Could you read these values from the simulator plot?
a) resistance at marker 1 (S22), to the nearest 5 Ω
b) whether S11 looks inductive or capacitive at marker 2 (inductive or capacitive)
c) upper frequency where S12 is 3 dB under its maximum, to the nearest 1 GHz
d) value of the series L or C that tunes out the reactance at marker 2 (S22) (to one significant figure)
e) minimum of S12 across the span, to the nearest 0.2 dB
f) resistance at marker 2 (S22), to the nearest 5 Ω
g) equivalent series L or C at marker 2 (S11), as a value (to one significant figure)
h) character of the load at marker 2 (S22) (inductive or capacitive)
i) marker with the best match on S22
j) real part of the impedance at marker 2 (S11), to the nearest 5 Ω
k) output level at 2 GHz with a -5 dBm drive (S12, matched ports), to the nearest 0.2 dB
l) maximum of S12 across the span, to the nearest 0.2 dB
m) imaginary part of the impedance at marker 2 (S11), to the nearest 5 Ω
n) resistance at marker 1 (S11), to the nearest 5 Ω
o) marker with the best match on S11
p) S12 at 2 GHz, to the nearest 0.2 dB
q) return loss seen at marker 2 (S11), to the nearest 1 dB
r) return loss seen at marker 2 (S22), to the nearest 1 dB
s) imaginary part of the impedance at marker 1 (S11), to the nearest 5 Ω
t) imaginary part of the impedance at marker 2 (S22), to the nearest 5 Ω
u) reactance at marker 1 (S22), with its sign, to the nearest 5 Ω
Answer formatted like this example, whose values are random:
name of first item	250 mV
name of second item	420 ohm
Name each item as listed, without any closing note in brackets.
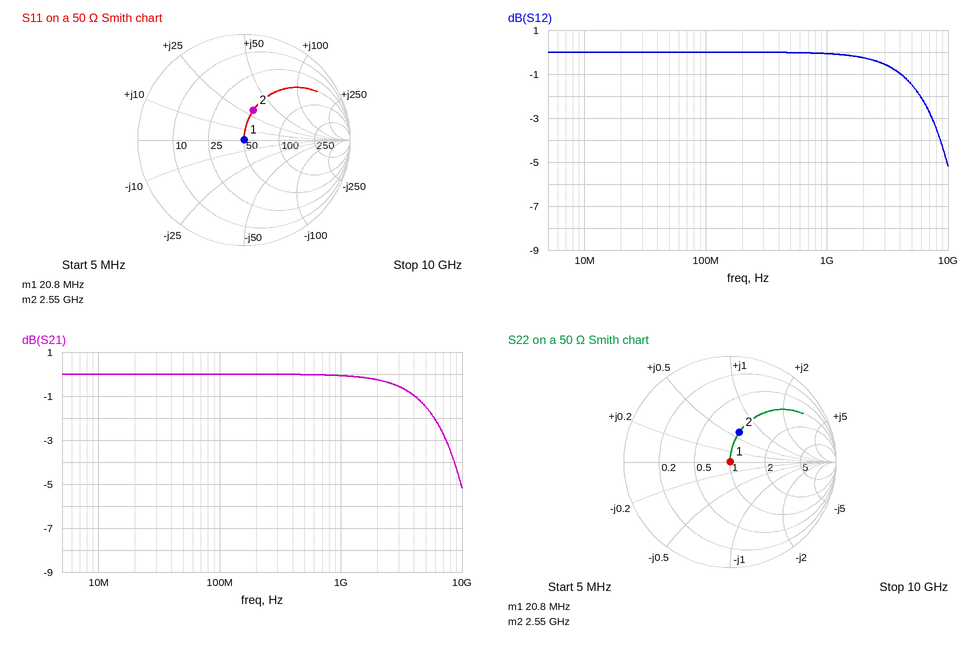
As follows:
resistance at marker 1 (S22), to the nearest 5 Ω	50 Ω
whether S11 looks inductive or capacitive at marker 2	inductive
upper frequency where S12 is 3 dB under its maximum, to the nearest 1 GHz	7 GHz
value of the series L or C that tunes out the reactance at marker 2 (S22)	2 pF
minimum of S12 across the span, to the nearest 0.2 dB	-5.2 dB
resistance at marker 2 (S22), to the nearest 5 Ω	50 Ω
equivalent series L or C at marker 2 (S11), as a value	2 nH
character of the load at marker 2 (S22)	inductive
marker with the best match on S22	marker 1
real part of the impedance at marker 2 (S11), to the nearest 5 Ω	50 Ω
output level at 2 GHz with a -5 dBm drive (S12, matched ports), to the nearest 0.2 dB	-5.2 dBm
maximum of S12 across the span, to the nearest 0.2 dB	0.0 dB
imaginary part of the impedance at marker 2 (S11), to the nearest 5 Ω	+30 Ω
resistance at marker 1 (S11), to the nearest 5 Ω	50 Ω
marker with the best match on S11	marker 1
S12 at 2 GHz, to the nearest 0.2 dB	-0.2 dB
return loss seen at marker 2 (S11), to the nearest 1 dB	11 dB
return loss seen at marker 2 (S22), to the nearest 1 dB	11 dB
imaginary part of the impedance at marker 1 (S11), to the nearest 5 Ω	0 Ω
imaginary part of the impedance at marker 2 (S22), to the nearest 5 Ω	+30 Ω
reactance at marker 1 (S22), with its sign, to the nearest 5 Ω	0 Ω
